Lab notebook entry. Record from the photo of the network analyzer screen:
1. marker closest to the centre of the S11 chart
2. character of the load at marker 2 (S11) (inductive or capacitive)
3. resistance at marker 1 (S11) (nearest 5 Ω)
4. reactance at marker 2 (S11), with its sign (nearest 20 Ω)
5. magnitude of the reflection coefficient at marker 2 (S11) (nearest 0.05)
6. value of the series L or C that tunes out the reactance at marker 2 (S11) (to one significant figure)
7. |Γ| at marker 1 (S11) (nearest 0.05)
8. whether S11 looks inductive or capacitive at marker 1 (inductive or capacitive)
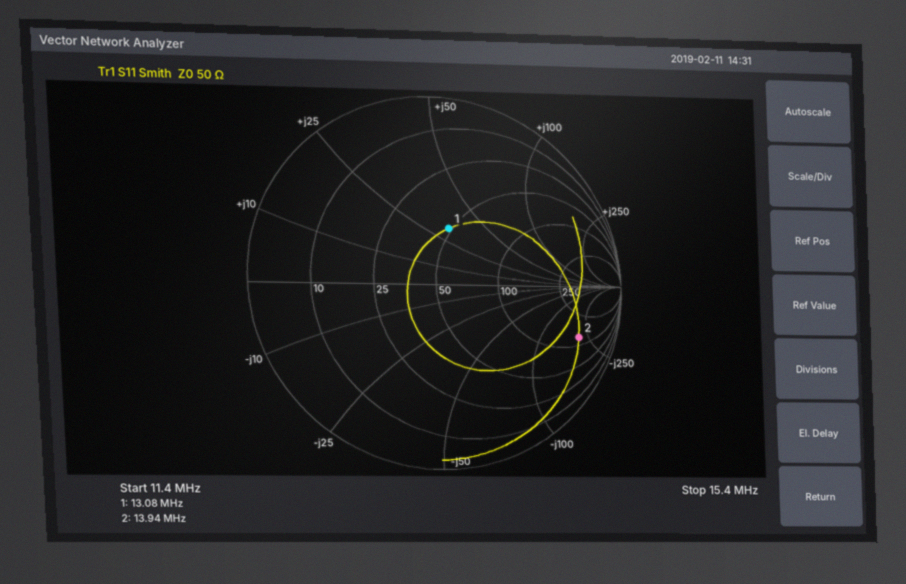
marker 1
capacitive
50 Ω
-200 Ω
0.80
2 µH
0.30
inductive
